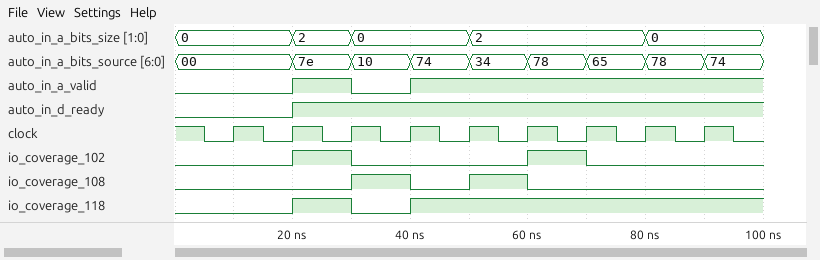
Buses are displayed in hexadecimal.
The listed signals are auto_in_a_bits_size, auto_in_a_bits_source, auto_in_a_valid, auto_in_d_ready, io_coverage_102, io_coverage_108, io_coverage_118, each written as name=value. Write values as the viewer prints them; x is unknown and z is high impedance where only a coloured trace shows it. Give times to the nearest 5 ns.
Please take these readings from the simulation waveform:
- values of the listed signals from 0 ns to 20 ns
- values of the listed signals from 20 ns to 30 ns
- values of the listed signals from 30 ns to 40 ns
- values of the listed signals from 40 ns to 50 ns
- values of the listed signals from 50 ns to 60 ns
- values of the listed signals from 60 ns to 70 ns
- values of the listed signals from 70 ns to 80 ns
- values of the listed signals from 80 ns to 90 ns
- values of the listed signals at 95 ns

auto_in_a_bits_size=0, auto_in_a_bits_source=00, auto_in_a_valid=0, auto_in_d_ready=0, io_coverage_102=0, io_coverage_108=0, io_coverage_118=0
auto_in_a_bits_size=2, auto_in_a_bits_source=7e, auto_in_a_valid=1, auto_in_d_ready=1, io_coverage_102=1, io_coverage_108=0, io_coverage_118=1
auto_in_a_bits_size=0, auto_in_a_bits_source=10, auto_in_a_valid=0, auto_in_d_ready=1, io_coverage_102=0, io_coverage_108=1, io_coverage_118=0
auto_in_a_bits_size=0, auto_in_a_bits_source=74, auto_in_a_valid=1, auto_in_d_ready=1, io_coverage_102=0, io_coverage_108=0, io_coverage_118=1
auto_in_a_bits_size=2, auto_in_a_bits_source=34, auto_in_a_valid=1, auto_in_d_ready=1, io_coverage_102=0, io_coverage_108=1, io_coverage_118=1
auto_in_a_bits_size=2, auto_in_a_bits_source=78, auto_in_a_valid=1, auto_in_d_ready=1, io_coverage_102=1, io_coverage_108=0, io_coverage_118=1
auto_in_a_bits_size=2, auto_in_a_bits_source=65, auto_in_a_valid=1, auto_in_d_ready=1, io_coverage_102=0, io_coverage_108=0, io_coverage_118=1
auto_in_a_bits_size=0, auto_in_a_bits_source=78, auto_in_a_valid=1, auto_in_d_ready=1, io_coverage_102=0, io_coverage_108=0, io_coverage_118=1
auto_in_a_bits_size=0, auto_in_a_bits_source=74, auto_in_a_valid=1, auto_in_d_ready=1, io_coverage_102=0, io_coverage_108=0, io_coverage_118=1
